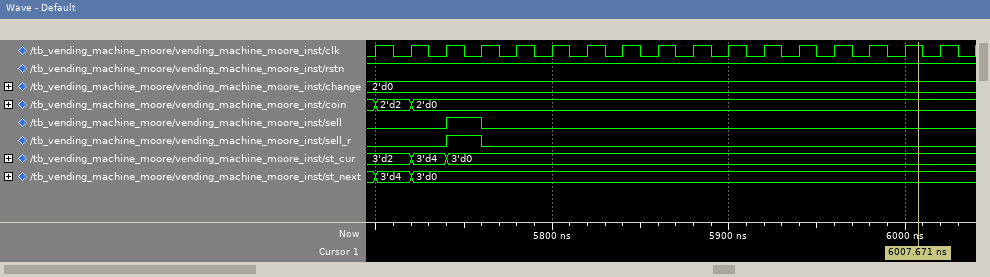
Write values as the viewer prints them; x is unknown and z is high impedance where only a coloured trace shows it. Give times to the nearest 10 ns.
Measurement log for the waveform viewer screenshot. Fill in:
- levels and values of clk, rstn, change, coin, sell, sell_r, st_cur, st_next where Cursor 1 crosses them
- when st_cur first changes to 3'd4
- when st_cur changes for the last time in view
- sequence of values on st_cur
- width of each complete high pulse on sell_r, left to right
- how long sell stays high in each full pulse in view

clk=1, rstn=1, change=2'd0, coin=2'd0, sell=0, sell_r=0, st_cur=3'd0, st_next=3'd0
5720 ns
5740 ns
3'd2, 3'd4, 3'd0
20 ns
20 ns
